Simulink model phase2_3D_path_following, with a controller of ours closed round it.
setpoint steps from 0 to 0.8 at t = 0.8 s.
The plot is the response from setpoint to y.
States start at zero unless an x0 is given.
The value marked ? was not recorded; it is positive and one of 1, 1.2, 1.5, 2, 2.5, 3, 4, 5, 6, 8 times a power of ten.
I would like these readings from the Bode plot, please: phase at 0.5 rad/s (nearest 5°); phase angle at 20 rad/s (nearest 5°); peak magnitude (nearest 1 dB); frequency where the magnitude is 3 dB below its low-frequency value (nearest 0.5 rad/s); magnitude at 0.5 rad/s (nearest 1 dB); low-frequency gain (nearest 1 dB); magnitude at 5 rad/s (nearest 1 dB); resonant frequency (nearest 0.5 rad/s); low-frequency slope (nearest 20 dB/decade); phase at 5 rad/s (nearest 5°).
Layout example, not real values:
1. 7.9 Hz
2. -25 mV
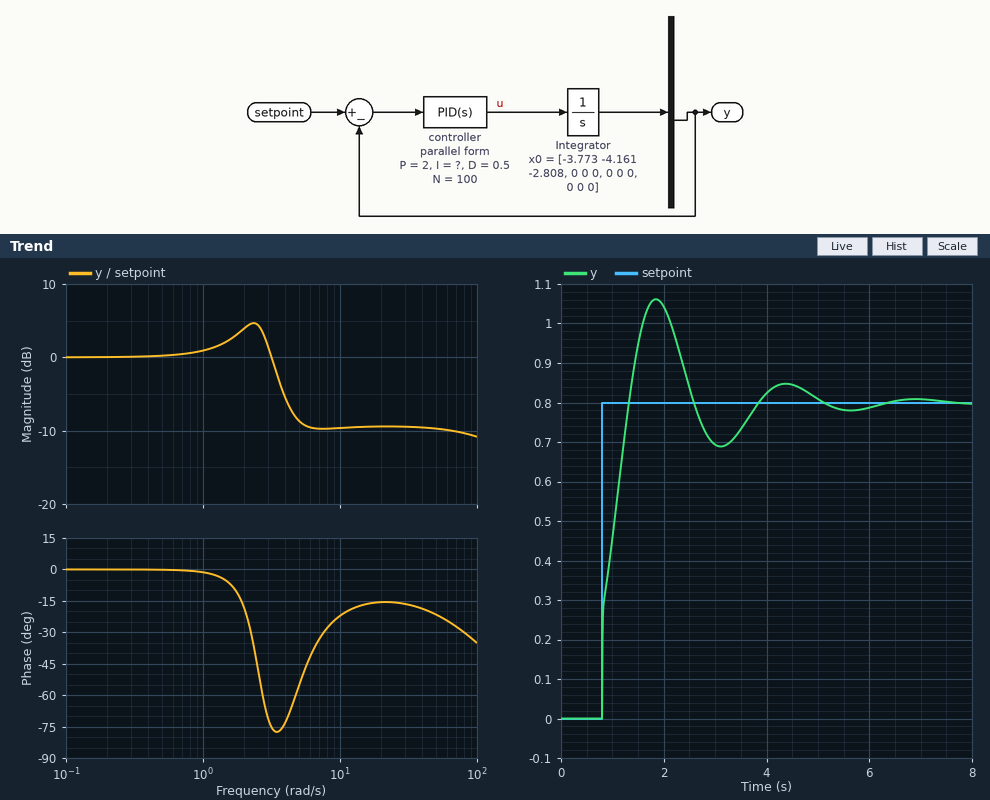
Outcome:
1. 0°
2. -15°
3. 5 dB
4. 3.5 rad/s
5. 0 dB
6. 0 dB
7. -9 dB
8. 2.5 rad/s
9. 0 dB/decade
10. -55°
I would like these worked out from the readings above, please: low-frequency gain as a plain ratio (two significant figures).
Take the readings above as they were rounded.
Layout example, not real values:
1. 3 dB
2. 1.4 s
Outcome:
1. 1.0
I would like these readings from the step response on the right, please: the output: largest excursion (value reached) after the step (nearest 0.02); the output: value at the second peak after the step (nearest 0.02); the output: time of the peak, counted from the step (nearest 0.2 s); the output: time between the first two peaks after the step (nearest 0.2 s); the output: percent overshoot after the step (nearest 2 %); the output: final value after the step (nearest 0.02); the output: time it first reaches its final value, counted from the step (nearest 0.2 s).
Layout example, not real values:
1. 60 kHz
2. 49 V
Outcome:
1. 1.06
2. 0.84
3. 1.0 s
4. 2.6 s
5. 32 %
6. 0.80
7. 0.6 s
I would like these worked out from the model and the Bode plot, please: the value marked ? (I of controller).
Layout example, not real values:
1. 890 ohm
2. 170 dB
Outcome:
1. 10
